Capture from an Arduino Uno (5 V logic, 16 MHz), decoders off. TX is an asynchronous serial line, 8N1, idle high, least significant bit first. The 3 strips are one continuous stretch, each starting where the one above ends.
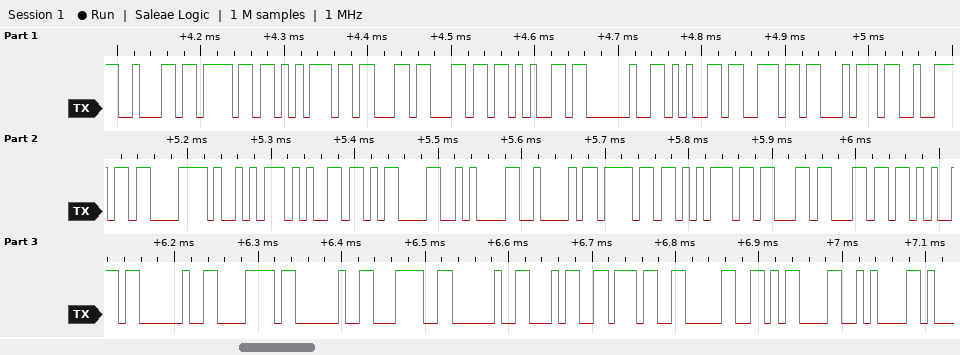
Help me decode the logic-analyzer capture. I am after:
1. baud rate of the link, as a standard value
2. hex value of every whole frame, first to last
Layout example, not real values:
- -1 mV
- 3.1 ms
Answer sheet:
- 115200 baud
- 0x62 0x6F 0x75 0x63 0x6C 0x65 0x20 0x65 0x6E 0x74 0x72 0xC3 0xA9 0x65 0x0D 0x0A 0x42 0x6F 0x75 0x63 0x6C 0x65 0x20 0x78 0x20 0x3C 0x20 0x34 0x37 0x30 0x0D 0x0A
